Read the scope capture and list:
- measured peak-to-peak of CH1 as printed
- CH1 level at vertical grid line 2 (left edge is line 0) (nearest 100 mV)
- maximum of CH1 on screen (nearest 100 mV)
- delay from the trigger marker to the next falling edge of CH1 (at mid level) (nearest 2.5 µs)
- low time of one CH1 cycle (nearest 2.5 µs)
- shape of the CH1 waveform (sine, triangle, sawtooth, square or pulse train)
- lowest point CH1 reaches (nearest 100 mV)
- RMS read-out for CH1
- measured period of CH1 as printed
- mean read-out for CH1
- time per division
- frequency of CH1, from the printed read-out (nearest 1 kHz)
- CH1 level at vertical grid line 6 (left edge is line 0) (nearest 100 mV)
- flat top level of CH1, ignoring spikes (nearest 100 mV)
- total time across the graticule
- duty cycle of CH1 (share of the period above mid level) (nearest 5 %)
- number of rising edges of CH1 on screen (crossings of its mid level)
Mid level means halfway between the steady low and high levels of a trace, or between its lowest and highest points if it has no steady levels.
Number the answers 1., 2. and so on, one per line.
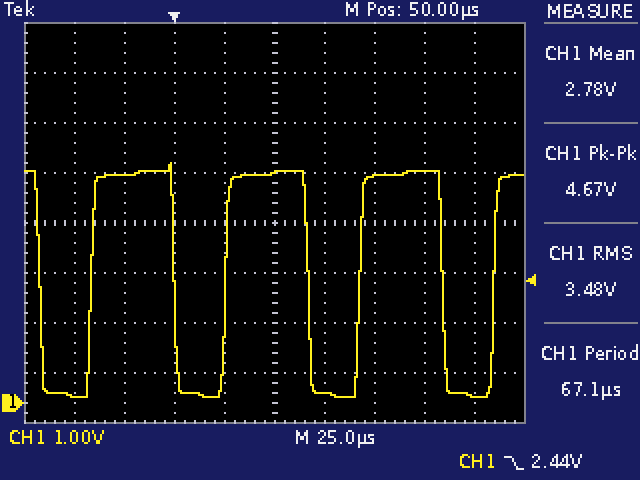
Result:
1. 4.67 V
2. 4.6 V
3. 4.8 V
4. 67.5 µs
5. 25.0 µs
6. pulse train
7. 100 mV
8. 3.48 V
9. 67.1 µs
10. 2.78 V
11. 25 µs
12. 15 kHz
13. 200 mV
14. 4.6 V
15. 250 µs
16. 60 %
17. 4
